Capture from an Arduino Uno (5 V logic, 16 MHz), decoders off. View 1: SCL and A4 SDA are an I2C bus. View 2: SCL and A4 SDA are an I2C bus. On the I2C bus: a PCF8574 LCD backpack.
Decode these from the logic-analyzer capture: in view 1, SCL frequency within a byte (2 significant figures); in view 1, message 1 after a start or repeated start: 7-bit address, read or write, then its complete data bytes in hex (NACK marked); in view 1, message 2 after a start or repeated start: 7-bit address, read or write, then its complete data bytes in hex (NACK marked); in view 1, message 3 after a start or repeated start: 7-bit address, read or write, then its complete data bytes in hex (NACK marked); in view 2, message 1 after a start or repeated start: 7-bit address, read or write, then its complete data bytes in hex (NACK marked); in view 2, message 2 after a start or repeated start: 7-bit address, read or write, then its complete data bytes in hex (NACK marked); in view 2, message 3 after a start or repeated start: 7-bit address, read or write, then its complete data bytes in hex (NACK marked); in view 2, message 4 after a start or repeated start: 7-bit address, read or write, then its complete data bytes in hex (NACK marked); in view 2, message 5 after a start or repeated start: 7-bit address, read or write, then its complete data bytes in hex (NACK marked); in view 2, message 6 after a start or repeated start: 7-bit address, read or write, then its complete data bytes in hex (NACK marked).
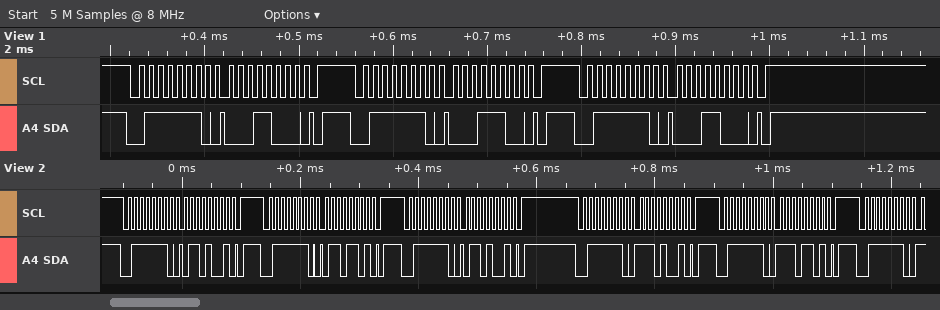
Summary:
100 kHz
0x3F write: 18
0x3F write: 1C
0x3F write: 18
0x3F write: 69
0x3F write: 6D
0x3F write: 69
0x3F write: E9
0x3F write: ED
0x3F write
